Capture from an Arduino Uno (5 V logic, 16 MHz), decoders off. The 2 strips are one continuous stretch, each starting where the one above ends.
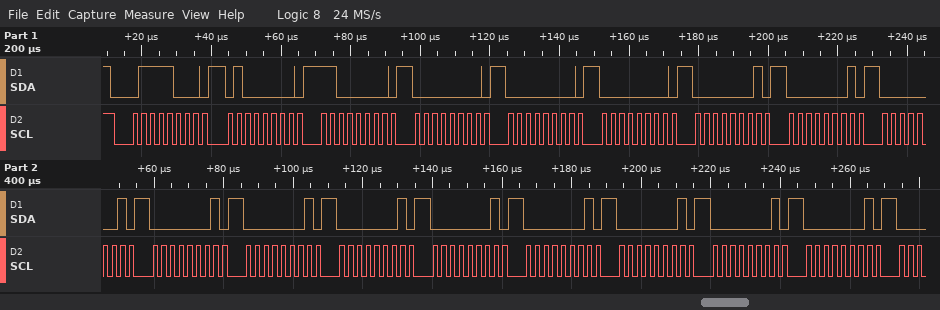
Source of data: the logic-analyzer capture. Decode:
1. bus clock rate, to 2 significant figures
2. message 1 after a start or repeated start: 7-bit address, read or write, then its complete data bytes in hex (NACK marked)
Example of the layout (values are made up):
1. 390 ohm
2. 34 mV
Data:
1. 400 kHz
2. 0x3C write: 40 C0 00 00 00 01 01 01 01 01 01 01 01 01 01 01
